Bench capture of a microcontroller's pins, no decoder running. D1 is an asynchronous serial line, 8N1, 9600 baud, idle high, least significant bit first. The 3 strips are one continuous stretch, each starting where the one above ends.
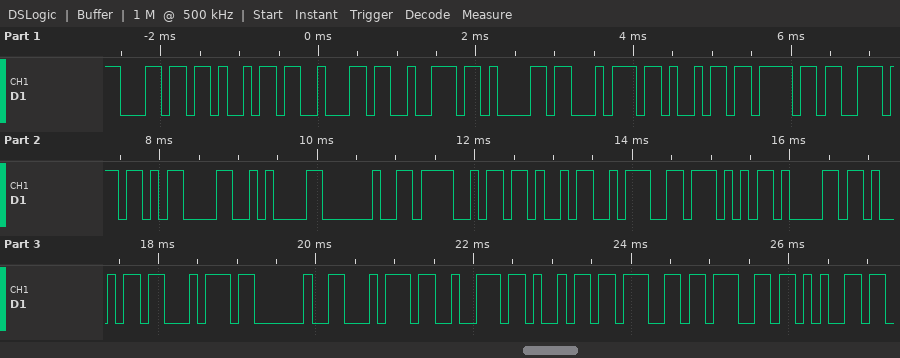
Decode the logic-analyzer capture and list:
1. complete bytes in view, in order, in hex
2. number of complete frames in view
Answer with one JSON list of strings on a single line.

["6C 69 62 72 61 74 69 6F 6E 0D 0A 20 4F 4B 3A 57 61 69 74 20 74 72 69 67 67 65", "26"]
